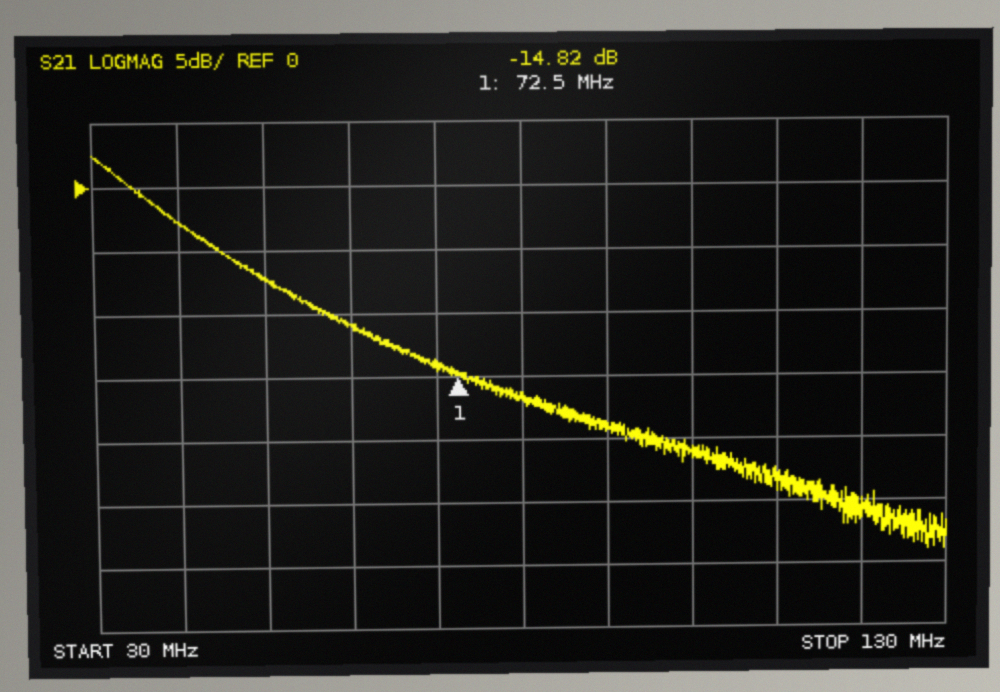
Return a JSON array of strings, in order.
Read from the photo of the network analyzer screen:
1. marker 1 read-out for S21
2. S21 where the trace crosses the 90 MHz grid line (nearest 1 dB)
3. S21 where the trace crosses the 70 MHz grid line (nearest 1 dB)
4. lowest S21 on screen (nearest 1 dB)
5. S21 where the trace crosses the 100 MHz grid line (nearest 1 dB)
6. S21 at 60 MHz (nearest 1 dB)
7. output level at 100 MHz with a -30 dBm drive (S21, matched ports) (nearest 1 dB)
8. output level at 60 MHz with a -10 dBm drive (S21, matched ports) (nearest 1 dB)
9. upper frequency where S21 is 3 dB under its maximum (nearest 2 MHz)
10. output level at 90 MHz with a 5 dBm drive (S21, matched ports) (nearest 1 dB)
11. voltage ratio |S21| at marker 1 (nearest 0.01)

["-14.82 dB", "-19 dB", "-14 dB", "-29 dB", "-21 dB", "-11 dB", "-51 dBm", "-21 dBm", "36 MHz", "-14 dBm", "0.18"]
